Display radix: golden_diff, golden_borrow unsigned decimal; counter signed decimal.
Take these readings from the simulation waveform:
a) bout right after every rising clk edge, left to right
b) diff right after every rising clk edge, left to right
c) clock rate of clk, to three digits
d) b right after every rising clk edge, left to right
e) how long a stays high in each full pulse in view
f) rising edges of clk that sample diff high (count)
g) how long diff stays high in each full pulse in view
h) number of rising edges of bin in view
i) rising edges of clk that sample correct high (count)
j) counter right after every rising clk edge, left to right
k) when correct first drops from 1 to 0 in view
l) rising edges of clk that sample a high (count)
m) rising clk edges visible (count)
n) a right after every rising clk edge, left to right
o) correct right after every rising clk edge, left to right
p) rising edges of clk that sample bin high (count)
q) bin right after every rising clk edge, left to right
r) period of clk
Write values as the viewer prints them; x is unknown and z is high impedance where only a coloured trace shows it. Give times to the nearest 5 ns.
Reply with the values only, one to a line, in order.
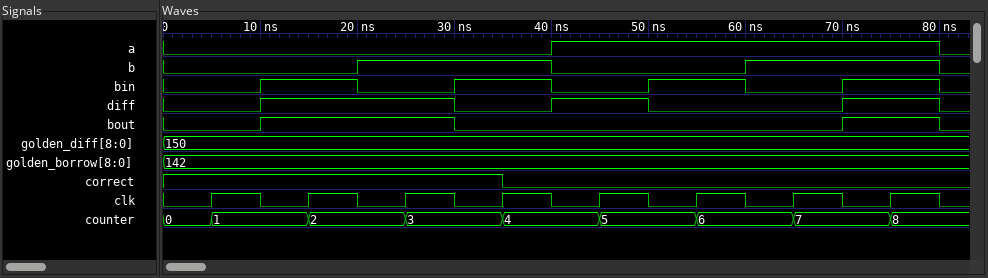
0 1 1 0 0 0 0 1
0 1 1 0 1 0 0 1
100 MHz
0 0 1 1 0 0 1 1
40 ns
4
20 ns, 10 ns, 10 ns
4
4
1, 2, 3, 4, 5, 6, 7, 8
35 ns
4
8
0 0 0 0 1 1 1 1
1 1 1 0 0 0 0 0
4
0 1 0 1 0 1 0 1
10 ns
